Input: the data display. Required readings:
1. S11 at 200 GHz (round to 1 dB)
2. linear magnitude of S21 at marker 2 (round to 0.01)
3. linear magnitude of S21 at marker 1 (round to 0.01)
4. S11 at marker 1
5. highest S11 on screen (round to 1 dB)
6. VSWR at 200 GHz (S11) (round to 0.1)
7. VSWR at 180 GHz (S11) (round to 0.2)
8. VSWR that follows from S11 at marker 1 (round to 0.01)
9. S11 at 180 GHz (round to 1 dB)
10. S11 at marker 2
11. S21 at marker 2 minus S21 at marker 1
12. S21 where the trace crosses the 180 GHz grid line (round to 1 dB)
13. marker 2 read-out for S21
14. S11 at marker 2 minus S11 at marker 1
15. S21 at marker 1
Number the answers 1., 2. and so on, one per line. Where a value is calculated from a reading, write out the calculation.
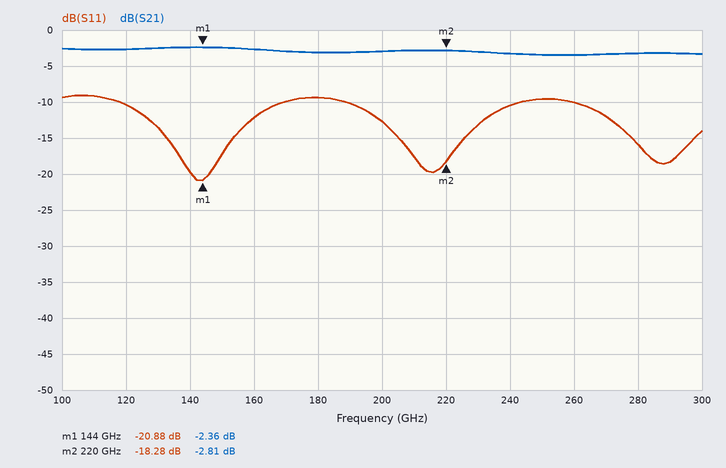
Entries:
1. -13 dB
2. 10^(-2.81/20) ≈ 0.72
3. 10^(-2.36/20) ≈ 0.76
4. -20.88 dB
5. -9 dB
6. |Γ| = 10^(-13/20) = 0.2239; VSWR = (1 + 0.2239)/(1 − 0.2239) ≈ 1.6
7. |Γ| = 10^(-9/20) = 0.3548; VSWR = (1 + 0.3548)/(1 − 0.3548) ≈ 2.10, so 2.0 to the nearest 0.2
8. (1 + 0.0904)/(1 − 0.0904) ≈ 1.20
9. -9 dB
10. -18.28 dB
11. -2.81 − (-2.36) = -0.45 dB
12. -3 dB
13. -2.81 dB
14. -18.28 − (-20.88) = 2.60 dB
15. -2.36 dB
